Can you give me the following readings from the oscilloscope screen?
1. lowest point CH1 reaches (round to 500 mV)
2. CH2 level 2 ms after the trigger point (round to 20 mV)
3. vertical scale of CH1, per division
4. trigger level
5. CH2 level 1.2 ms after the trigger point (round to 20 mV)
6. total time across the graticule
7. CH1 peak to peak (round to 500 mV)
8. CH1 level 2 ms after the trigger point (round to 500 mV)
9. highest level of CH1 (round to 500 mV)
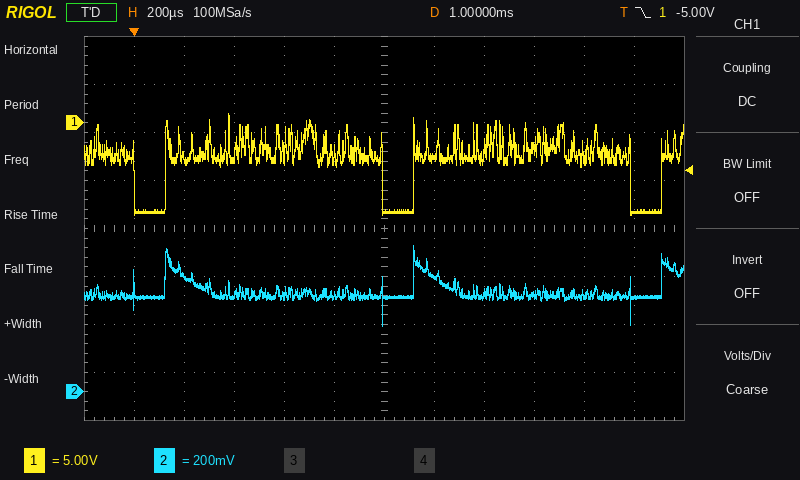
-9.5 V
400 mV
5 V
-5.00 V
480 mV
2.4 ms
10.5 V
-9.5 V
1.0 V
